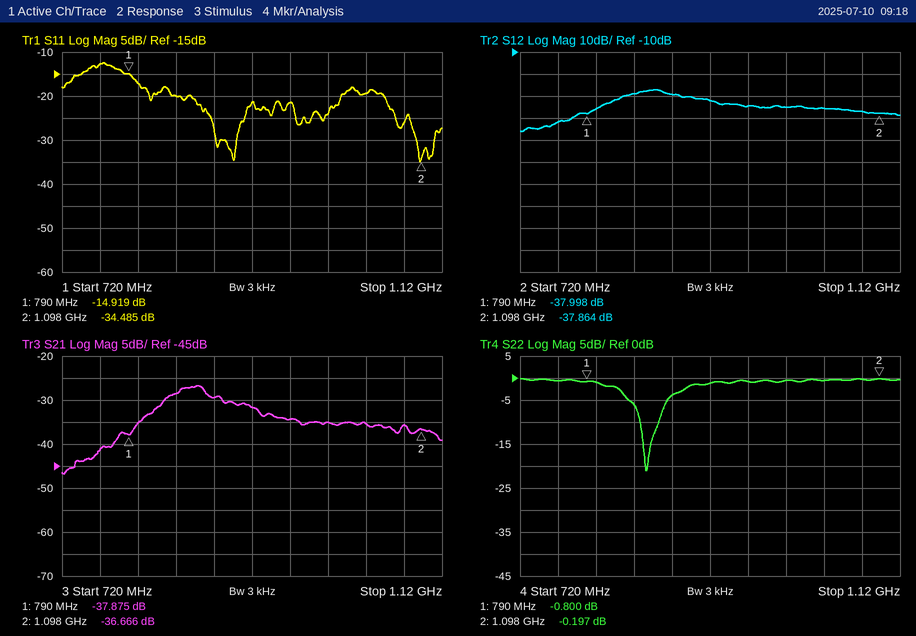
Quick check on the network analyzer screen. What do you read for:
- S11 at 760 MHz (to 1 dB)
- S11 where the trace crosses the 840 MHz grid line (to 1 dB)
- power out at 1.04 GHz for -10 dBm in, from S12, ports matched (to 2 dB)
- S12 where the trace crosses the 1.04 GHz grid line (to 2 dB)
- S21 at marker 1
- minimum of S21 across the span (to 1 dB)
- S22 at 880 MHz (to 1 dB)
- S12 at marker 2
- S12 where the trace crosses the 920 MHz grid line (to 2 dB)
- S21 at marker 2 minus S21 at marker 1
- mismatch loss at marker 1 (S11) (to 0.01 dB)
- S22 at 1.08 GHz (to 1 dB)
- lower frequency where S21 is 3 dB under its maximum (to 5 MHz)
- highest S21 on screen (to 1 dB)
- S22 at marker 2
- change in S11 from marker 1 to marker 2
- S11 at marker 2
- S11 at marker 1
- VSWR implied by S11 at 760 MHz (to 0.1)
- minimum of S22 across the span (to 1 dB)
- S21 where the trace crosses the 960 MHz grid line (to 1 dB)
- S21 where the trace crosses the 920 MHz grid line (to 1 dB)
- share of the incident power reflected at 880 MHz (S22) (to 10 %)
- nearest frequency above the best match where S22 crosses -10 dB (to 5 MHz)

-13 dB
-20 dB
-46 dBm
-36 dB
-37.875 dB
-47 dB
-4 dB
-37.864 dB
-32 dB
1.209 dB
0.14 dB
0 dB
830 MHz
-27 dB
-0.197 dB
-19.566 dB
-34.485 dB
-14.919 dB
1.6
-21 dB
-34 dB
-32 dB
40 %
865 MHz
